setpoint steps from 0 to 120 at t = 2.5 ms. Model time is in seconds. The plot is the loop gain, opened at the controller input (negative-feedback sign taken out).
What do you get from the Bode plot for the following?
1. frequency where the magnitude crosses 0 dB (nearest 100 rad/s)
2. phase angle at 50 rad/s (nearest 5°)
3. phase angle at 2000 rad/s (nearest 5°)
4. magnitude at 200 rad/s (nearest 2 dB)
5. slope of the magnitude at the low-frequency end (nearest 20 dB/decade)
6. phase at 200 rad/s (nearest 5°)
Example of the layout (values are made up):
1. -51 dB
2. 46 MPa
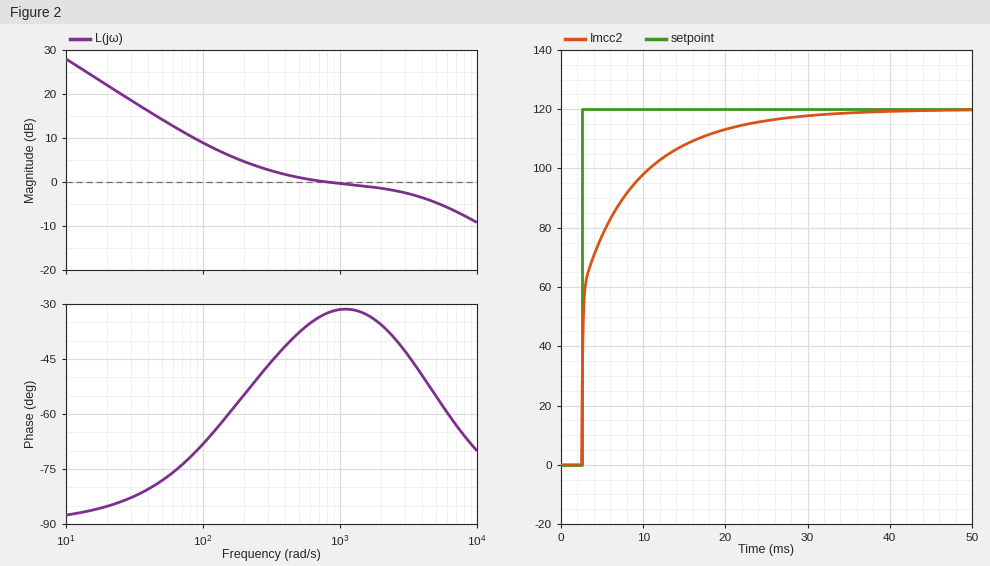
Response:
1. 800 rad/s
2. -80°
3. -35°
4. 4 dB
5. -20 dB/decade
6. -55°
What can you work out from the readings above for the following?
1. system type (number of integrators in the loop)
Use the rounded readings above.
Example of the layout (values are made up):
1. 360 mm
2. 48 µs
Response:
1. 1
